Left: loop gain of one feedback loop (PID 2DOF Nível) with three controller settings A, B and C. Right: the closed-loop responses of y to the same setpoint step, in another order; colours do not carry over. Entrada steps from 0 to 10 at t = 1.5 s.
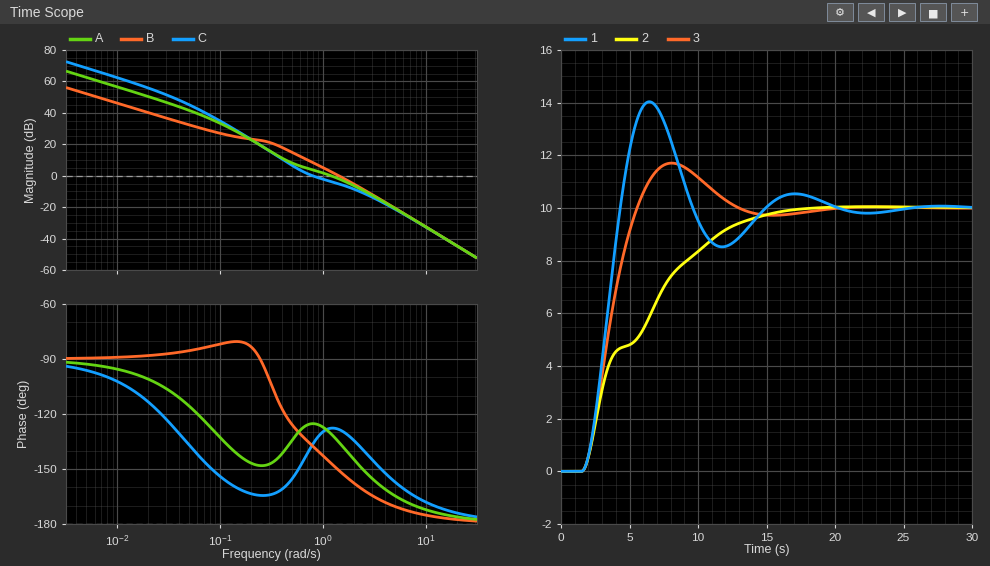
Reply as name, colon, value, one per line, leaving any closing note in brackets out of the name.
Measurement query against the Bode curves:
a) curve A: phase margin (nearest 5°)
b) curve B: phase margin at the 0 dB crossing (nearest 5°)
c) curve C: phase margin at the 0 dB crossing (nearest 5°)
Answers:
curve A: phase margin: 50°
curve B: phase margin at the 0 dB crossing: 30°
curve C: phase margin at the 0 dB crossing: 45°
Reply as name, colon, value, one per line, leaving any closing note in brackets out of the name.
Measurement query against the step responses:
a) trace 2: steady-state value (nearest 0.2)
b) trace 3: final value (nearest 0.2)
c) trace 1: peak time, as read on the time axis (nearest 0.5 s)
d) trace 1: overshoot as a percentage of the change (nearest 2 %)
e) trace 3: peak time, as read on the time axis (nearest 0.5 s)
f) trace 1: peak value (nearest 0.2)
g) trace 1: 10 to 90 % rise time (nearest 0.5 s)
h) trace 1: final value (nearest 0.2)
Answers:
trace 2: steady-state value: 10.0
trace 3: final value: 10.0
trace 1: peak time, as read on the time axis: 6.5 s
trace 1: overshoot as a percentage of the change: 40 %
trace 3: peak time, as read on the time axis: 8.0 s
trace 1: peak value: 14.0
trace 1: 10 to 90 % rise time: 2.0 s
trace 1: final value: 10.0
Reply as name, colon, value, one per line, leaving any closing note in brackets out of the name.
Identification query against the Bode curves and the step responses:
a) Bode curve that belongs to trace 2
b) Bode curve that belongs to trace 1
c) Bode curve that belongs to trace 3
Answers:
Bode curve that belongs to trace 2: B
Bode curve that belongs to trace 1: C
Bode curve that belongs to trace 3: A
